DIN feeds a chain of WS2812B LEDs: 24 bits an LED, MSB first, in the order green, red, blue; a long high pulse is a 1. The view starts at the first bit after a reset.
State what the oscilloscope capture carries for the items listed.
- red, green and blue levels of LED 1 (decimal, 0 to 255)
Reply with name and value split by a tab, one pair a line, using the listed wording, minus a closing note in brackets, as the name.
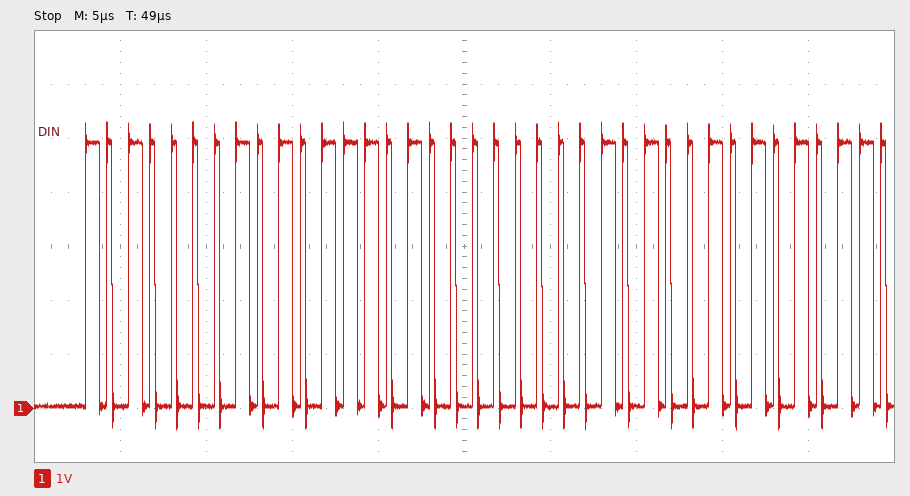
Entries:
red, green and blue levels of LED 1	93, 161, 0
